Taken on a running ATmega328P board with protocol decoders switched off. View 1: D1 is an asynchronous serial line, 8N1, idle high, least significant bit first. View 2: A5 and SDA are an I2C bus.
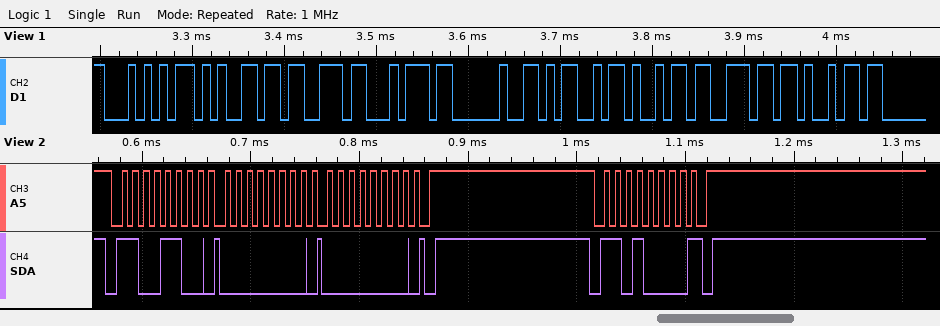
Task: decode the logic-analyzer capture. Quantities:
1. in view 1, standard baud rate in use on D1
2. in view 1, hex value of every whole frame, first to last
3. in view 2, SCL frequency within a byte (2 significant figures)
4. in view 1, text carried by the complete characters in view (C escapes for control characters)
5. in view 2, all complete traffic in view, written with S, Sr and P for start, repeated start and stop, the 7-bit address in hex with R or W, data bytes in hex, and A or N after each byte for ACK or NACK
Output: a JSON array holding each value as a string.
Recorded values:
["115200 baud", "0x54 0x65 0x73 0x74 0x20 0x4D 0x69 0x6E 0x69", "100 kHz", "\"Test Mini\"", "S 66W A 00 A 00 A P S 68W N P"]
